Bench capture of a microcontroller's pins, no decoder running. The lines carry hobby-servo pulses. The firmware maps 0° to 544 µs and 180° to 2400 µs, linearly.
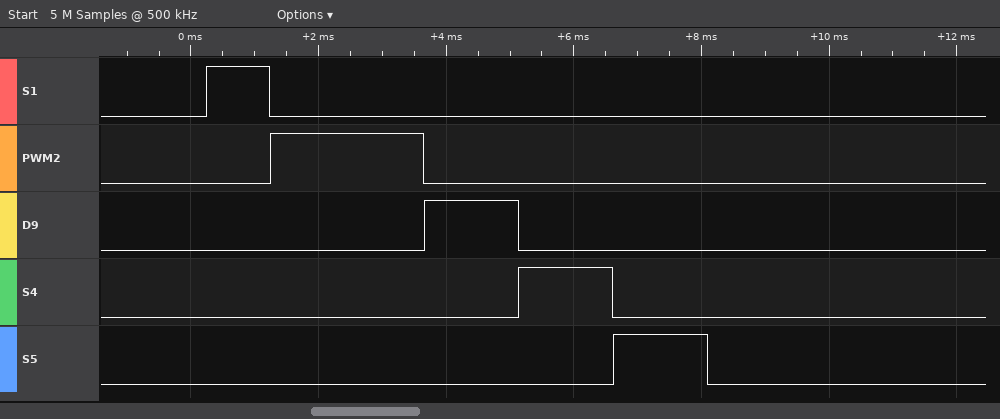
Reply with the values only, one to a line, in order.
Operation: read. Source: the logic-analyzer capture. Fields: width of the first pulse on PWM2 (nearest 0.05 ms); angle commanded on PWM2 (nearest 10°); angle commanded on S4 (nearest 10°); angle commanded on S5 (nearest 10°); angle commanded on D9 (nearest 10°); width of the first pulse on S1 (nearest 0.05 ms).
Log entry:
2.40 ms
180°
90°
90°
90°
1.00 ms
